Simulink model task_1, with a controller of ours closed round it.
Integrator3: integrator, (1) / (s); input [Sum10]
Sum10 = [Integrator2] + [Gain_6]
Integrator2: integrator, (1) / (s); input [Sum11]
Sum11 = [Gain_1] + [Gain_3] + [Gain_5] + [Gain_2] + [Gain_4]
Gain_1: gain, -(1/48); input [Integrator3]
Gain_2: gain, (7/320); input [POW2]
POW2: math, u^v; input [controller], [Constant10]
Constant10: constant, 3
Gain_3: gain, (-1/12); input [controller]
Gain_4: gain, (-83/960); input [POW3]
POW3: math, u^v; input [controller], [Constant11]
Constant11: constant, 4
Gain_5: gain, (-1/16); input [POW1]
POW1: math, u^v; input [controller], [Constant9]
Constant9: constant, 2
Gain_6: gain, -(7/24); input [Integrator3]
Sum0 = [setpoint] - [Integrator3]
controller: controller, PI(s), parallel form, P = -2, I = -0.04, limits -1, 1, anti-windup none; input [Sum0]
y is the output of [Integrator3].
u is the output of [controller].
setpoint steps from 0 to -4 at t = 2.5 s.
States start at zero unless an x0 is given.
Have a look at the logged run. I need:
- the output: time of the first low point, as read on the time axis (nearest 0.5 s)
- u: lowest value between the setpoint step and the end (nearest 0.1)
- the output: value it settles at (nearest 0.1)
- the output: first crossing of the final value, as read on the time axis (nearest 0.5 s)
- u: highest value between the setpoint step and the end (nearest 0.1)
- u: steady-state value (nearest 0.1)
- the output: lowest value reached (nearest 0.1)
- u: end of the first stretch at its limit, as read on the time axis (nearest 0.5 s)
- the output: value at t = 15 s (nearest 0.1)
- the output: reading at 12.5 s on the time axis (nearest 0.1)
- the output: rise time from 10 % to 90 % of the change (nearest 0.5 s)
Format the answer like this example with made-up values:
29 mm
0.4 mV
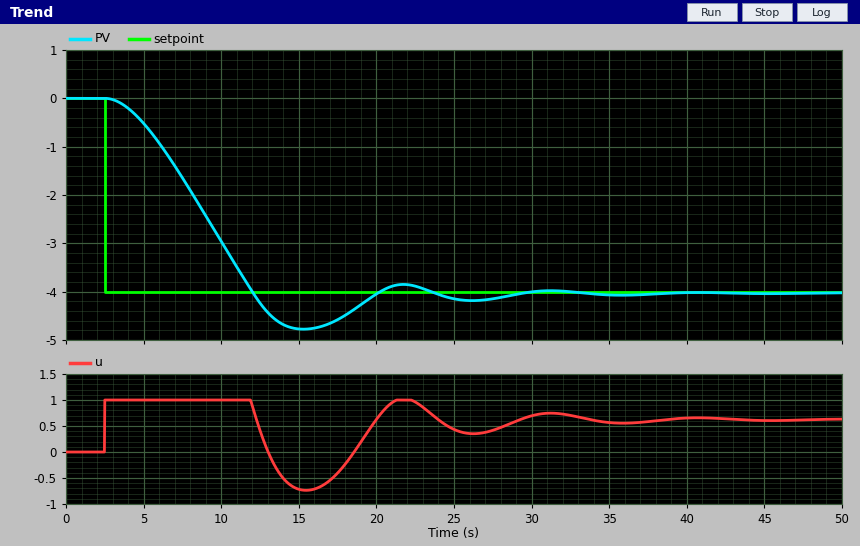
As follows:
15.5 s
-0.7
-4.0
12.0 s
1.0
0.6
-4.8
12.0 s
-4.8
-4.2
6.5 s
